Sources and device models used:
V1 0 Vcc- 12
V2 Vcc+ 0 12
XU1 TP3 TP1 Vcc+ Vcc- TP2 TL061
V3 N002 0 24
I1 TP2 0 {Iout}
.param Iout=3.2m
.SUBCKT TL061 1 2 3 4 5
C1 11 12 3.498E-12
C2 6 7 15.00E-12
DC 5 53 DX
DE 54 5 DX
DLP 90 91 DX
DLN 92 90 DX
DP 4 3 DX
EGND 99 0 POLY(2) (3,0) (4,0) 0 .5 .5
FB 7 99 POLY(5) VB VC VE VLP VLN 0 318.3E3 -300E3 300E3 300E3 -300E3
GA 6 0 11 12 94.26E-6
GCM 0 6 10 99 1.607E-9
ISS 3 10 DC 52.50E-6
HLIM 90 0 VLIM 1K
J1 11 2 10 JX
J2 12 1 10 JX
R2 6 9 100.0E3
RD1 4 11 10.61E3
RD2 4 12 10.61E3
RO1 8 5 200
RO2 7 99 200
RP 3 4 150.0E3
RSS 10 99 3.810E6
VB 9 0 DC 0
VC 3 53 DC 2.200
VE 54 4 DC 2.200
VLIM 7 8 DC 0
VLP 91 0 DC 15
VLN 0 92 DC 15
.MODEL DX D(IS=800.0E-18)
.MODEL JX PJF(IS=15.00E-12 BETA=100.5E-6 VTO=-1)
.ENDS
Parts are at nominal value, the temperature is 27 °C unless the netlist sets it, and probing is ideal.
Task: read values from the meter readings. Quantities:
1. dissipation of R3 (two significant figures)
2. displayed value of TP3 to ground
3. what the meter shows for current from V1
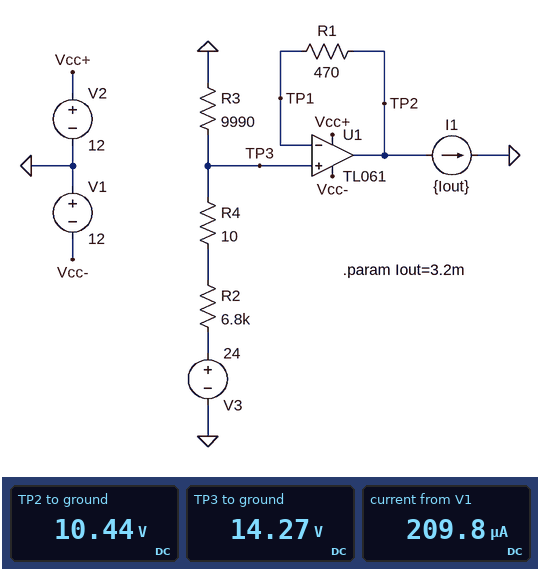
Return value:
20 mW
14.27 V
209.8 µA
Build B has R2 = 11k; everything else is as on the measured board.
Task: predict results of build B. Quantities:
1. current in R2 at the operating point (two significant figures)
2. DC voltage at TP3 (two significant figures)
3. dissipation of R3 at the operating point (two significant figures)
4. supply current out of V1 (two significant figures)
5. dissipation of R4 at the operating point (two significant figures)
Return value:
1.1 mA
11 V
13 mW
210 µA
13 µW
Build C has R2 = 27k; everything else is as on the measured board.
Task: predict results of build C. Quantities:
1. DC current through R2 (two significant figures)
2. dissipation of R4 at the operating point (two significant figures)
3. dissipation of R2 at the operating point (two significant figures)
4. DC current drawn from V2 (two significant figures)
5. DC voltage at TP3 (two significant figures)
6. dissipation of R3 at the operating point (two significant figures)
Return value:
650 µA
4.2 µW
11 mW
210 µA
6.5 V
4.2 mW
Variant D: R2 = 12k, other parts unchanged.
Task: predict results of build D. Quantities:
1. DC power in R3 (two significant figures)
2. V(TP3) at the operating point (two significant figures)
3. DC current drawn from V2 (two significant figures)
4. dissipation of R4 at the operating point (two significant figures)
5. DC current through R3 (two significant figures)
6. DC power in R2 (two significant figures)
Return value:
12 mW
11 V
170 µA
12 µW
1.1 mA
14 mW
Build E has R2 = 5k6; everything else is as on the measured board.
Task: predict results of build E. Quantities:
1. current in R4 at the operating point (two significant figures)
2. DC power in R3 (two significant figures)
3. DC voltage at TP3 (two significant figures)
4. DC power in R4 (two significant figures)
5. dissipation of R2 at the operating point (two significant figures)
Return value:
1.5 mA
24 mW
15 V
24 µW
13 mW
